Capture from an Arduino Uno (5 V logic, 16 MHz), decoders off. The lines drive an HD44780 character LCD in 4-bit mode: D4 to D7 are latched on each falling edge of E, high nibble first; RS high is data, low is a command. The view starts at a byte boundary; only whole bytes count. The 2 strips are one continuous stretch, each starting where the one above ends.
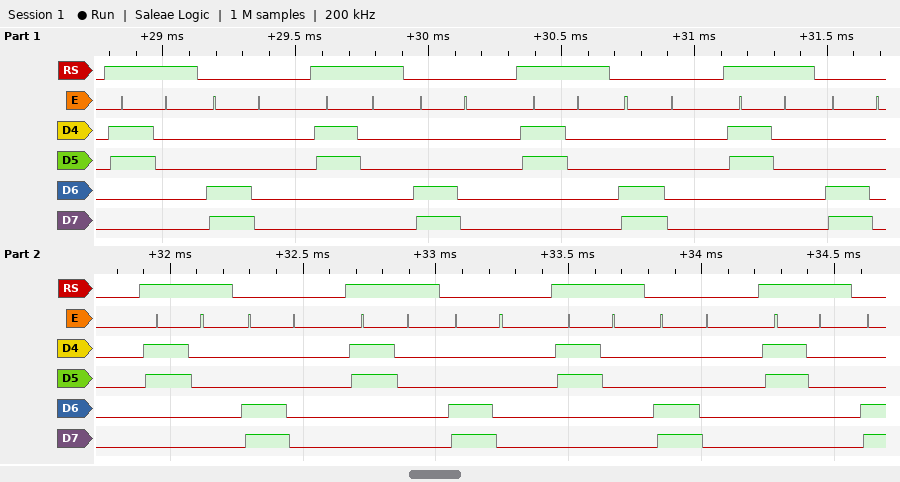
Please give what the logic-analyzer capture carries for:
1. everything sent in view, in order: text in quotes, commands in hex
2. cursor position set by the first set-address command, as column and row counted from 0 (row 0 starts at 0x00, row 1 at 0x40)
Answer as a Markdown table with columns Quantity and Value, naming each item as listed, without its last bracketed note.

| Quantity | Value |
|---|---|
| everything sent in view, in order: text in quotes, commands in hex | "0" 0xC0 "0" 0xC0 "0" 0xC0 "0" 0xC0 "0" 0xC0 "0" 0xC0 "0" 0xC0 "0" |
| cursor position set by the first set-address command, as column and row counted from 0 | column 0, row 1 |
